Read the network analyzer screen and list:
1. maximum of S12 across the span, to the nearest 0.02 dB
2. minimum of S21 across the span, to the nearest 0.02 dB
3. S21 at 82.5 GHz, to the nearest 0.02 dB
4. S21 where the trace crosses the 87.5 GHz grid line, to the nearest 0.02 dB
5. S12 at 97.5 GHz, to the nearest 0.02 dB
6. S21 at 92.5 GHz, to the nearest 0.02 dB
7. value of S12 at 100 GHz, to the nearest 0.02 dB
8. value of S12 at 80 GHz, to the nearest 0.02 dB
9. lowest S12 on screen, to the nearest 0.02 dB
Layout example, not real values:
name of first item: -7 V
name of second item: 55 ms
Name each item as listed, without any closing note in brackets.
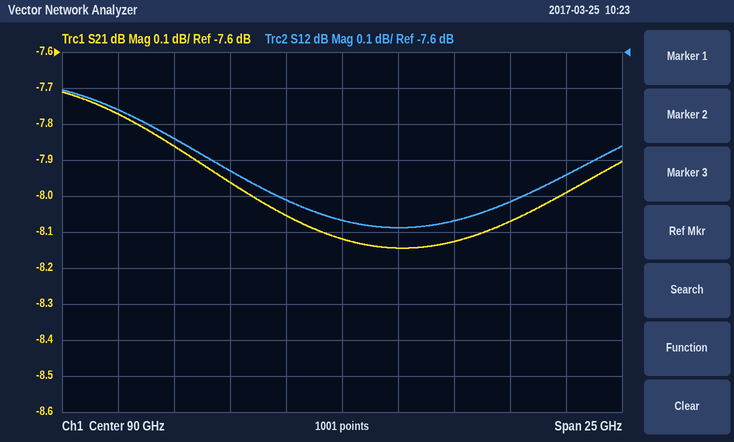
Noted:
maximum of S12 across the span, to the nearest 0.02 dB: -7.70 dB
minimum of S21 across the span, to the nearest 0.02 dB: -8.14 dB
S21 at 82.5 GHz, to the nearest 0.02 dB: -7.86 dB
S21 where the trace crosses the 87.5 GHz grid line, to the nearest 0.02 dB: -8.06 dB
S12 at 97.5 GHz, to the nearest 0.02 dB: -8.02 dB
S21 at 92.5 GHz, to the nearest 0.02 dB: -8.14 dB
value of S12 at 100 GHz, to the nearest 0.02 dB: -7.94 dB
value of S12 at 80 GHz, to the nearest 0.02 dB: -7.76 dB
lowest S12 on screen, to the nearest 0.02 dB: -8.08 dB
